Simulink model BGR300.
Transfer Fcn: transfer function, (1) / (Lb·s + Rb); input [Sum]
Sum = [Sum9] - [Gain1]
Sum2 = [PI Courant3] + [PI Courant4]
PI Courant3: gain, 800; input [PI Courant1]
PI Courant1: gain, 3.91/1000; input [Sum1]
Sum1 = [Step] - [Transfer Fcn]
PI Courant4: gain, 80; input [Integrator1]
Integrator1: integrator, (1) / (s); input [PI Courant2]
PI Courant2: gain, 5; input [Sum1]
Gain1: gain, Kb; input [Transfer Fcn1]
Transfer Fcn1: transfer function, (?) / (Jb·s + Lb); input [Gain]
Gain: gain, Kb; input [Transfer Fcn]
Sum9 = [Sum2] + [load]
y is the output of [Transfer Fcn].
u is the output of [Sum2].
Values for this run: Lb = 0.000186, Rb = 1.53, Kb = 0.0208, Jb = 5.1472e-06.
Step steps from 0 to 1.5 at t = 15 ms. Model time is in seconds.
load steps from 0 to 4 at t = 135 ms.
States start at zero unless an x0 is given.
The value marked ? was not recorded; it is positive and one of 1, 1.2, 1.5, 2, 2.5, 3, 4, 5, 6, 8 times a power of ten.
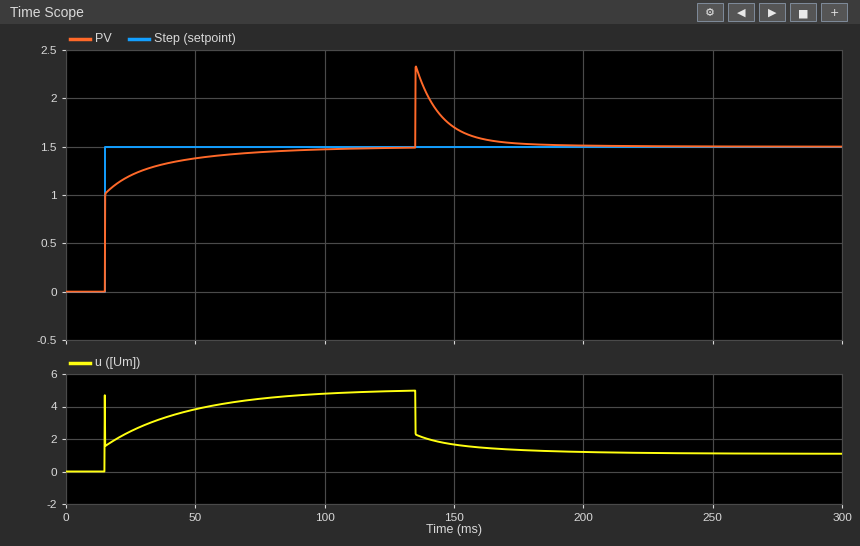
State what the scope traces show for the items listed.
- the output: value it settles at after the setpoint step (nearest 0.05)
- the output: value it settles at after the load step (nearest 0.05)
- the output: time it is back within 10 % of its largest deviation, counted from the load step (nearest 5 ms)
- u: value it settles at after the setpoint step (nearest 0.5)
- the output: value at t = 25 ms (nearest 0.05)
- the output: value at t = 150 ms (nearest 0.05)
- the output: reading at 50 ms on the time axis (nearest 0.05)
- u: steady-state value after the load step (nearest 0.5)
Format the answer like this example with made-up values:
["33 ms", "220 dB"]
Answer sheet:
["1.50", "1.50", "25 ms", "5.0", "1.20", "1.70", "1.40", "1.0"]
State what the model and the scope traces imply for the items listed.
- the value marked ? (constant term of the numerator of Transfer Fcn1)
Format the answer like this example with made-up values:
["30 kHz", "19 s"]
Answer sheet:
["0.8"]
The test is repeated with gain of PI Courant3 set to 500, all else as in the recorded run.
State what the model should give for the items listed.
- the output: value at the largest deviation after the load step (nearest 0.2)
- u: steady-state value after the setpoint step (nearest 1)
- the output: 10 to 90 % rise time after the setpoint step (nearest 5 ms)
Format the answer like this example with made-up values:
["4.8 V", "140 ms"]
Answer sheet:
["2.6", "5", "25 ms"]
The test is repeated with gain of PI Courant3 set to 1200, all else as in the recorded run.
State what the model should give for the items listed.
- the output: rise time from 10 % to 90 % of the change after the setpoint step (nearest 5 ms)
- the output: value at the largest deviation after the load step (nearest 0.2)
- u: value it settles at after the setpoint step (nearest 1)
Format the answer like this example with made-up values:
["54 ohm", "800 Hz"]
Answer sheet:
["30 ms", "2.2", "5"]
